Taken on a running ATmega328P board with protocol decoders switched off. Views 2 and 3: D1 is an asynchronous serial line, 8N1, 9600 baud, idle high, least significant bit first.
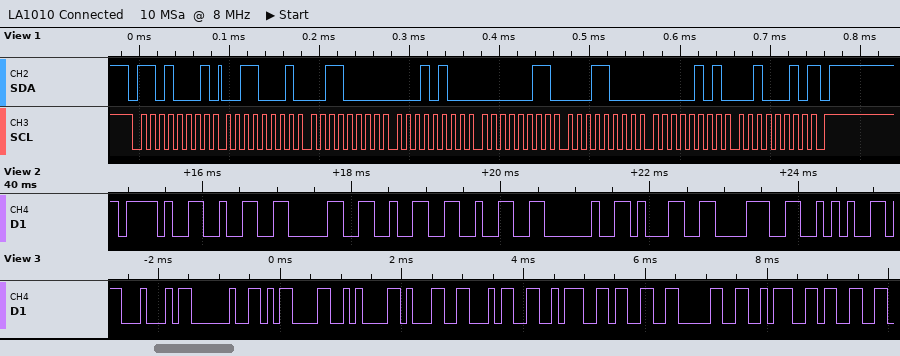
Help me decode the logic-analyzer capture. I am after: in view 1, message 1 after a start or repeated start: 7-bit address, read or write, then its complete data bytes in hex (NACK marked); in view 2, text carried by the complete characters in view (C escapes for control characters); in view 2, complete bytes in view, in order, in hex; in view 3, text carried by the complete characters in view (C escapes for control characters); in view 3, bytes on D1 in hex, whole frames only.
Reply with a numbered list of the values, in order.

1. 0x68 read: 31 30 14 03 18 05 22 NACK
2. "/2022 18*"
3. 2F 32 30 32 32 20 31 38 2A
4. "D \r\n14:30:3"
5. 44 20 0D 0A 31 34 3A 33 30 3A 33
